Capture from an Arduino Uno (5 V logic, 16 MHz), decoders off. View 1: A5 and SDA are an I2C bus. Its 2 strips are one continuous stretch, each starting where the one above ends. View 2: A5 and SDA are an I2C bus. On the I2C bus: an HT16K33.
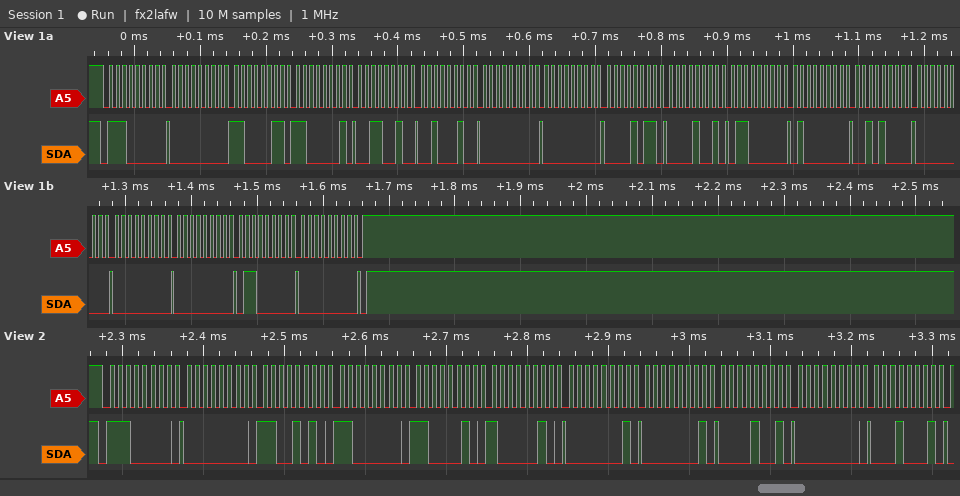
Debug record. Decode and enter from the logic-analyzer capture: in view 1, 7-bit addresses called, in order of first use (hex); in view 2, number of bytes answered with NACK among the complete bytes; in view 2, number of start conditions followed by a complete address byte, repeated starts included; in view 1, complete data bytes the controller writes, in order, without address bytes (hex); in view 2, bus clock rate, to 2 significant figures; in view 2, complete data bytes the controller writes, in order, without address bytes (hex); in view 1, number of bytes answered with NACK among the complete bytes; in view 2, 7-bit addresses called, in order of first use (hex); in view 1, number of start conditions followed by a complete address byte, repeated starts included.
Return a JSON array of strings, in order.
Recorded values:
["0x70", "0", "1", "00 C3 C1 32 22 00 00 0B 09 60 40 28 00 00 00 60 00", "100 kHz", "00 CA C0 C2 82 01 01 09 00 11", "0", "0x70", "1"]
